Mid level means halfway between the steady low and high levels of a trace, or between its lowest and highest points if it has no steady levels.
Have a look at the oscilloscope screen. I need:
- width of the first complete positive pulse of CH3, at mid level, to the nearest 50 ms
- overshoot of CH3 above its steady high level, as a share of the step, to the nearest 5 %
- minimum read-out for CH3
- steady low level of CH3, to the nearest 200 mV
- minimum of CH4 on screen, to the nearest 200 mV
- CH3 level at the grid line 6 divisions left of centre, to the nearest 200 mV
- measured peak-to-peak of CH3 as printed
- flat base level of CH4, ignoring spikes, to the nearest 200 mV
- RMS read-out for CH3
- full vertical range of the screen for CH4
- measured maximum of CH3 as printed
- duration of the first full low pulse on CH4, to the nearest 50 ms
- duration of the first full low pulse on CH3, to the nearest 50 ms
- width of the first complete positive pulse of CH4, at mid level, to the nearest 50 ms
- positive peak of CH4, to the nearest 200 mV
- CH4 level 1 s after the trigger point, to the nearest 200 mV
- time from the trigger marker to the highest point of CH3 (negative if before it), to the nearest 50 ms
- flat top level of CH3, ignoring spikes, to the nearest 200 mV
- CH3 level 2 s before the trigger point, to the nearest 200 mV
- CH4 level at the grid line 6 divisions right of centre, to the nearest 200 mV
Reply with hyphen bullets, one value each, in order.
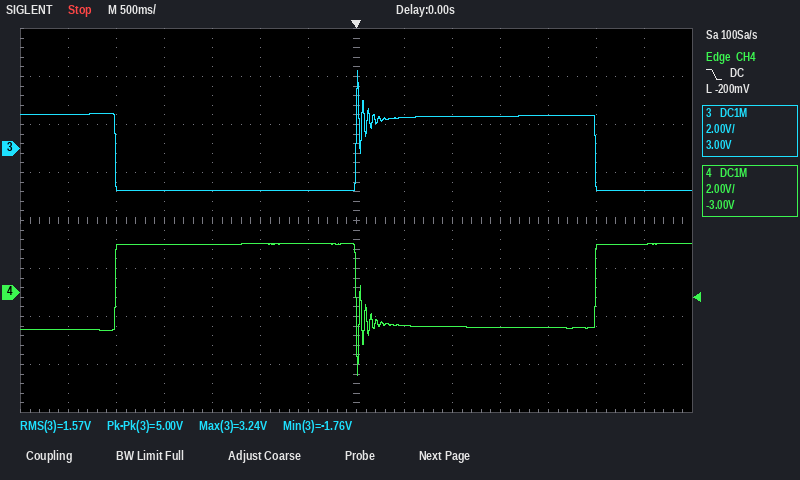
- 2.50 s
- 60 %
- -1.76 V
- -1.8 V
- -3.4 V
- 1.4 V
- 5.00 V
- -1.4 V
- 1.57 V
- 16 V
- 3.24 V
- 2.50 s
- 2.50 s
- 2.50 s
- 2.0 V
- -1.4 V
- 0 ms
- 1.4 V
- -1.8 V
- 2.0 V
